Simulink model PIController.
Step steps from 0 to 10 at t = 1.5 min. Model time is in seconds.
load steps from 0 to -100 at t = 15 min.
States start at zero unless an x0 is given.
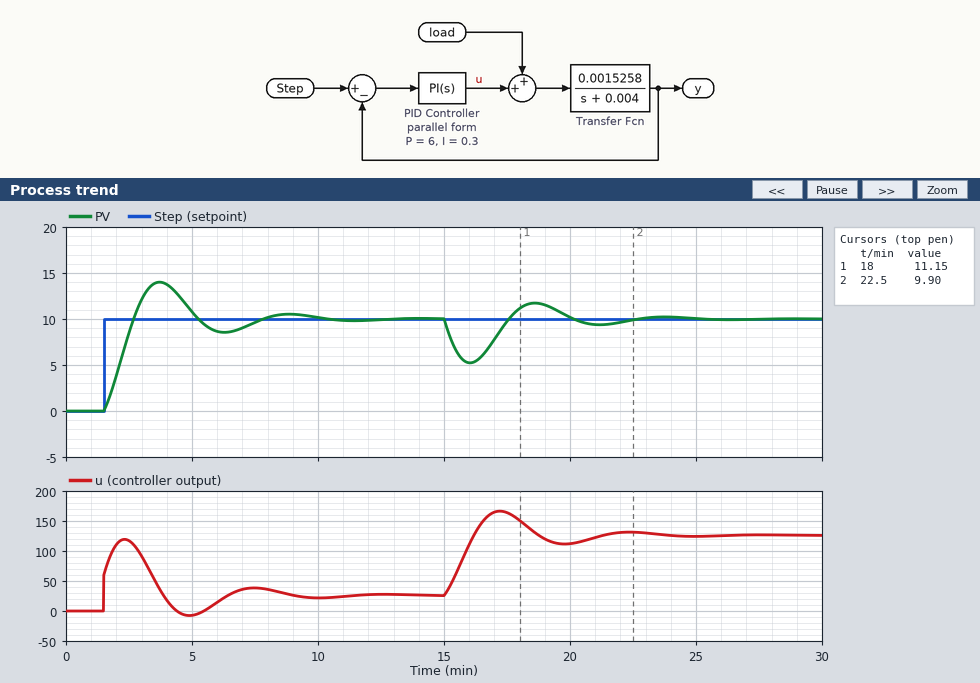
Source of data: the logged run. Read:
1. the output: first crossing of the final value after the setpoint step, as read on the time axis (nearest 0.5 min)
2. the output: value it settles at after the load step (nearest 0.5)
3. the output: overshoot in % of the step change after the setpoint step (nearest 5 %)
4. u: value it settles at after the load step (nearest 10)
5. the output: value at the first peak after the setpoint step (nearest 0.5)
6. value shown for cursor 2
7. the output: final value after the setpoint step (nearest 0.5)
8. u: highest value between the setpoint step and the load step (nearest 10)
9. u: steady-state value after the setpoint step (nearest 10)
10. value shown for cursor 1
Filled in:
2.5 min
10.0
40 %
130
14.0
9.90
10.0
120
30
11.15
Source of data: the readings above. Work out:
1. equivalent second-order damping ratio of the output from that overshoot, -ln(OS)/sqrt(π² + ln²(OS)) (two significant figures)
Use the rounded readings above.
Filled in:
0.28
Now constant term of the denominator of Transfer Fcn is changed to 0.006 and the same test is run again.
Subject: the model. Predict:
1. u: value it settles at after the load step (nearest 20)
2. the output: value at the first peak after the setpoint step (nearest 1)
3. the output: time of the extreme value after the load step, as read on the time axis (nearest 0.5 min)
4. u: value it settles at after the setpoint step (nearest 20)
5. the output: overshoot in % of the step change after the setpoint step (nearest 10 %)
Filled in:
140
13
16.0 min
40
30 %
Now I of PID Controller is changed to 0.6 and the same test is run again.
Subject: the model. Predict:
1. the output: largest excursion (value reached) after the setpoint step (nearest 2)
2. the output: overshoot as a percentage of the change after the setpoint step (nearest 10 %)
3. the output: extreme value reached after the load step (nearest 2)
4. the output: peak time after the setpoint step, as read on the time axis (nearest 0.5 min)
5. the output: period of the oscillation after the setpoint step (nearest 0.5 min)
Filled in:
16
50 %
6
3.0 min
3.5 min
